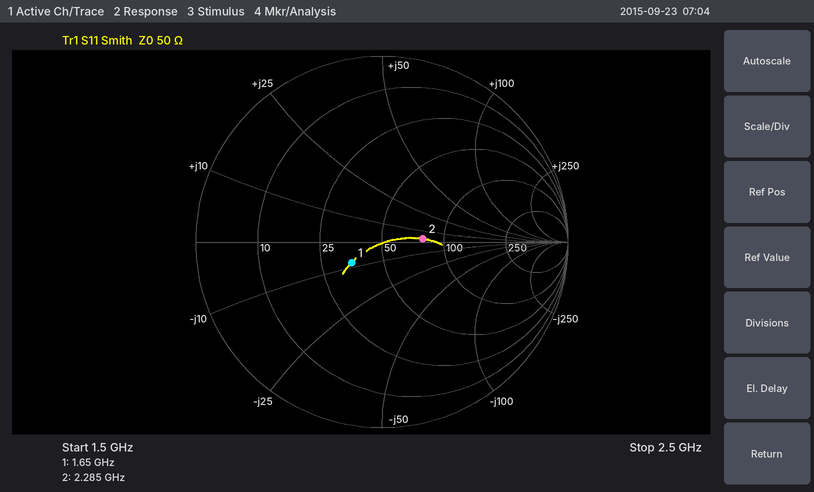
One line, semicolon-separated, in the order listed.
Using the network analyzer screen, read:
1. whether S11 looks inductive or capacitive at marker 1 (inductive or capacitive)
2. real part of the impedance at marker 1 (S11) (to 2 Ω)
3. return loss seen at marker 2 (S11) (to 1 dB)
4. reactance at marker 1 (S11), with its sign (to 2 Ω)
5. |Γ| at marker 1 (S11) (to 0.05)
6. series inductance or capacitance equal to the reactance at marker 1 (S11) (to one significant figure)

capacitive; 36 Ω; 13 dB; -8 Ω; 0.20; 10 pF
